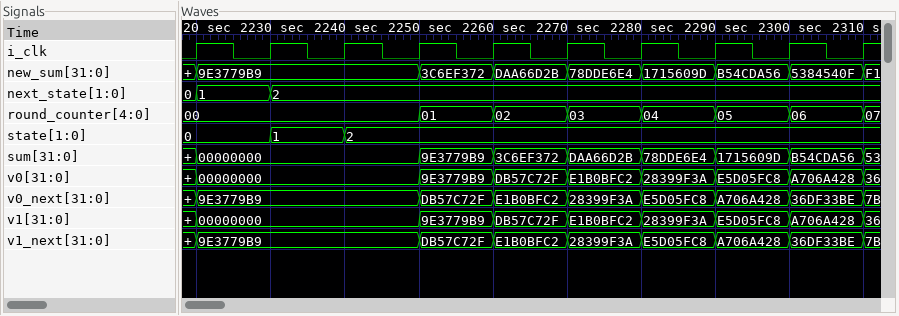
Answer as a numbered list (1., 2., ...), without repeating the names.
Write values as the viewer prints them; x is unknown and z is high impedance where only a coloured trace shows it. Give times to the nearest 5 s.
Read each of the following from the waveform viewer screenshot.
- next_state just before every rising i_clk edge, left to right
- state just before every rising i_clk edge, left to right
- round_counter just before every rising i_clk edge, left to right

1. 0, 1, 2, 2, 2, 2, 2, 2, 2, 2
2. 0, 0, 1, 2, 2, 2, 2, 2, 2, 2
3. 00, 00, 00, 00, 01, 02, 03, 04, 05, 06
